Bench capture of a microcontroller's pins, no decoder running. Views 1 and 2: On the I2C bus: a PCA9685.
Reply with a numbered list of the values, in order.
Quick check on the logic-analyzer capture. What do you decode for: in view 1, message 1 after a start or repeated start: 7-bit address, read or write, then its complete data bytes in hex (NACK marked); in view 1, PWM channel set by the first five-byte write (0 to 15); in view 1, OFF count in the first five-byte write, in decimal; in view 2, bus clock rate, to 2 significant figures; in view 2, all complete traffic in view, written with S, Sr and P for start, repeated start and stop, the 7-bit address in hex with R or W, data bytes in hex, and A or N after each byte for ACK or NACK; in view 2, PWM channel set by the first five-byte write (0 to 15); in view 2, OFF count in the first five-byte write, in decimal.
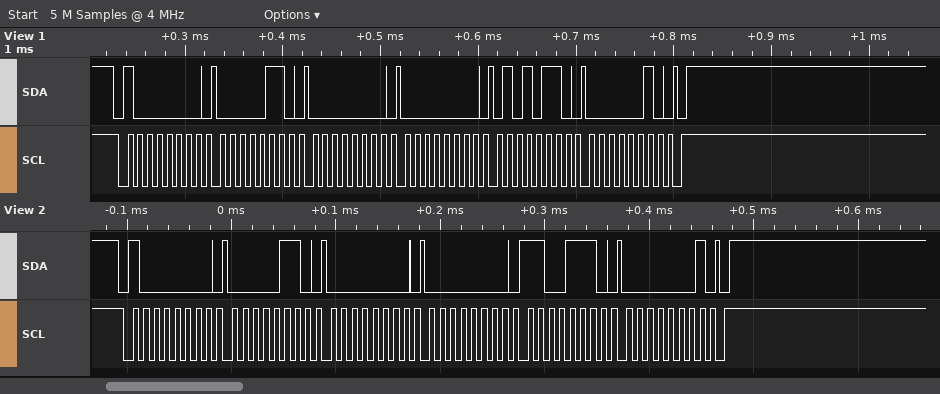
1. 0x40 write: 06 00 00 56 02
2. 0
3. 598
4. 100 kHz
5. S 40W A 06 A 00 A 00 A CE A 01 A P
6. 0
7. 462
